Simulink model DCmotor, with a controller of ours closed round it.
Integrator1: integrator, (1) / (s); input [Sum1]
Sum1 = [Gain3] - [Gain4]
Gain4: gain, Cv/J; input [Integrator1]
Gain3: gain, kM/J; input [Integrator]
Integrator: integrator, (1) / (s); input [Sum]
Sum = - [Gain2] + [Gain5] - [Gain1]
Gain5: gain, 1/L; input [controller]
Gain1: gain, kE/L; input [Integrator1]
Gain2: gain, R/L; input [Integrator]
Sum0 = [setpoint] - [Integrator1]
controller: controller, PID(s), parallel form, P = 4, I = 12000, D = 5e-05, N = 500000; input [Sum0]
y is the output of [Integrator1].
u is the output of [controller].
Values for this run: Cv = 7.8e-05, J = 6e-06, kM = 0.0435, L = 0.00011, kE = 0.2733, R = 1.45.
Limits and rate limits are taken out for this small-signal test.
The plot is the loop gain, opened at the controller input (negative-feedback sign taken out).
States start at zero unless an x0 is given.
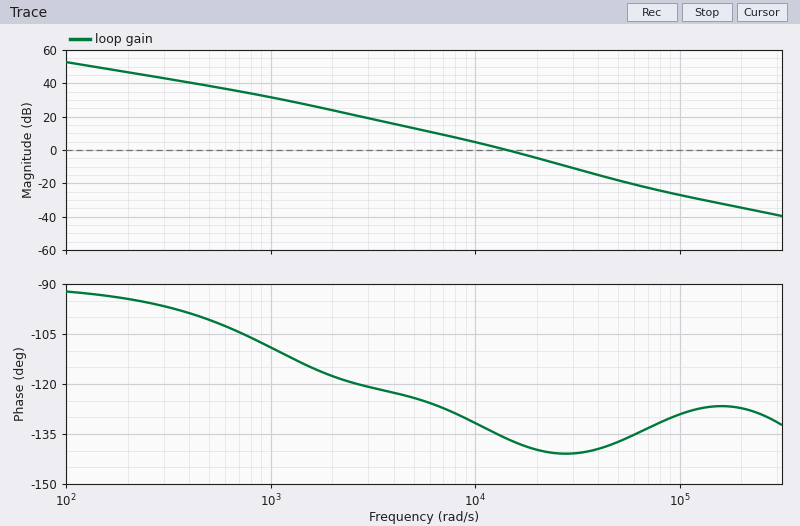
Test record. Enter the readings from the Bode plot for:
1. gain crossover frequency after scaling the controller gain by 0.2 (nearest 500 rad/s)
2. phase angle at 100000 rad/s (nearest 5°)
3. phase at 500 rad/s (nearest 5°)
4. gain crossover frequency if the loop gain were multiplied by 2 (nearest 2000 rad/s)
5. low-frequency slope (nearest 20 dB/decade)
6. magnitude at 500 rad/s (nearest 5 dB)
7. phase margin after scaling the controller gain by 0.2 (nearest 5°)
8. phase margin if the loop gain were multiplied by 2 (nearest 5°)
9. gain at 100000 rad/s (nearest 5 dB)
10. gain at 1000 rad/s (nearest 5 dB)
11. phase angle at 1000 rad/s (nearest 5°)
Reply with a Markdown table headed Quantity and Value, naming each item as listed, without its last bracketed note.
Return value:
| Quantity | Value |
|---|---|
| gain crossover frequency after scaling the controller gain by 0.2 | 4500 rad/s |
| phase angle at 100000 rad/s | -130° |
| phase at 500 rad/s | -100° |
| gain crossover frequency if the loop gain were multiplied by 2 | 22000 rad/s |
| low-frequency slope | -20 dB/decade |
| magnitude at 500 rad/s | 40 dB |
| phase margin after scaling the controller gain by 0.2 | 55° |
| phase margin if the loop gain were multiplied by 2 | 40° |
| gain at 100000 rad/s | -25 dB |
| gain at 1000 rad/s | 30 dB |
| phase angle at 1000 rad/s | -110° |
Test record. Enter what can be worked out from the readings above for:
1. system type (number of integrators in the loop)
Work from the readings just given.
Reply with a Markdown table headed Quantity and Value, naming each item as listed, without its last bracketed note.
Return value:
| Quantity | Value |
|---|---|
| system type | 1 |
